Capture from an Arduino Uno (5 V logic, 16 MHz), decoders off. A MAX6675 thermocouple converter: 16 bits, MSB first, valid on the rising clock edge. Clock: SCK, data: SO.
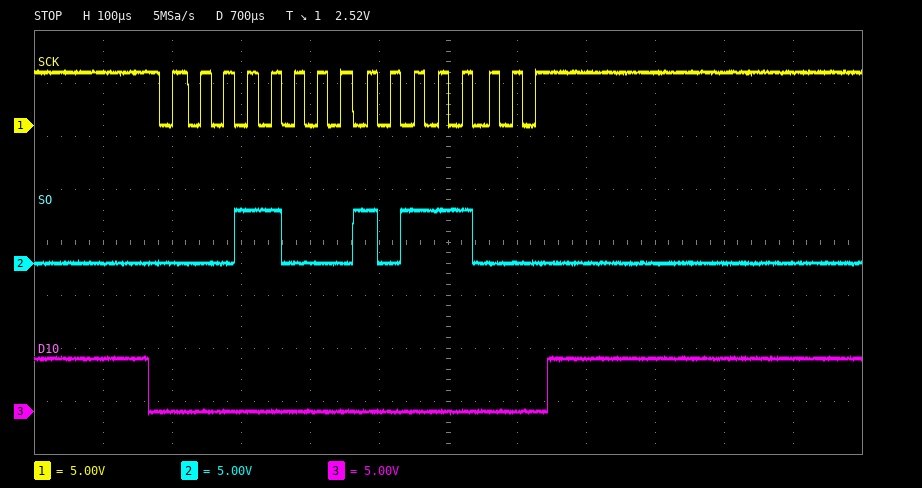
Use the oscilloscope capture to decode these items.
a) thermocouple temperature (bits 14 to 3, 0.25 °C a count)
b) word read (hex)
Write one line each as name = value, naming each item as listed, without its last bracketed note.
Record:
thermocouple temperature = 197.75 °C
word read = 0x18B8
